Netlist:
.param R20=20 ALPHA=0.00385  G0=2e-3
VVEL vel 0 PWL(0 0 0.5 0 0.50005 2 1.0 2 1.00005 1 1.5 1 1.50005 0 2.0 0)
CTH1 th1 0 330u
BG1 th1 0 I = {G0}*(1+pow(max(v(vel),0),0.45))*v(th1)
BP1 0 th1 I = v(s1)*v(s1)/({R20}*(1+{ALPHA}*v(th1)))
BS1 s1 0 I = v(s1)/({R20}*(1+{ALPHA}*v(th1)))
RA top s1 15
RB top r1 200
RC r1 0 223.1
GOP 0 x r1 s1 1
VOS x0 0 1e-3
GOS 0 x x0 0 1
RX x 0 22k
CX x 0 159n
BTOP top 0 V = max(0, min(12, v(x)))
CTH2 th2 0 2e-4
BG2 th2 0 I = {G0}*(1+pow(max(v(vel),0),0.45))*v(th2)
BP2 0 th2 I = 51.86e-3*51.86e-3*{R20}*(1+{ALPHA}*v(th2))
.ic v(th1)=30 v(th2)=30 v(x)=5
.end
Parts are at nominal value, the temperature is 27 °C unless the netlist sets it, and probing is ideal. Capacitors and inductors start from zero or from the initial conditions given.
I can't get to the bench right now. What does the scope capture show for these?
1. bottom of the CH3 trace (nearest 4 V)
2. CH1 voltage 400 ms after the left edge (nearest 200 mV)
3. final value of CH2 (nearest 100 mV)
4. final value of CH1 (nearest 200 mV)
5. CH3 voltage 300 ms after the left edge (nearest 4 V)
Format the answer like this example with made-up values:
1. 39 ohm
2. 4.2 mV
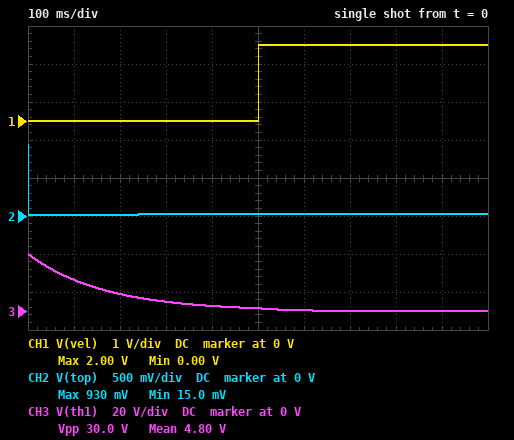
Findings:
1. 0 V
2. 0 V
3. 0 V
4. 2.0 V
5. 4 V
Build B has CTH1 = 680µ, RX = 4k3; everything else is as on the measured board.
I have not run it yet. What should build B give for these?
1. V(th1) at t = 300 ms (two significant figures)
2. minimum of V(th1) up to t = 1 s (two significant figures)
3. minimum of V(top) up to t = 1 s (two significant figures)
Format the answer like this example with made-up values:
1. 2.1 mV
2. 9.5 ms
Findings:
1. 12 V
2. 210 mV
3. 14 mV
